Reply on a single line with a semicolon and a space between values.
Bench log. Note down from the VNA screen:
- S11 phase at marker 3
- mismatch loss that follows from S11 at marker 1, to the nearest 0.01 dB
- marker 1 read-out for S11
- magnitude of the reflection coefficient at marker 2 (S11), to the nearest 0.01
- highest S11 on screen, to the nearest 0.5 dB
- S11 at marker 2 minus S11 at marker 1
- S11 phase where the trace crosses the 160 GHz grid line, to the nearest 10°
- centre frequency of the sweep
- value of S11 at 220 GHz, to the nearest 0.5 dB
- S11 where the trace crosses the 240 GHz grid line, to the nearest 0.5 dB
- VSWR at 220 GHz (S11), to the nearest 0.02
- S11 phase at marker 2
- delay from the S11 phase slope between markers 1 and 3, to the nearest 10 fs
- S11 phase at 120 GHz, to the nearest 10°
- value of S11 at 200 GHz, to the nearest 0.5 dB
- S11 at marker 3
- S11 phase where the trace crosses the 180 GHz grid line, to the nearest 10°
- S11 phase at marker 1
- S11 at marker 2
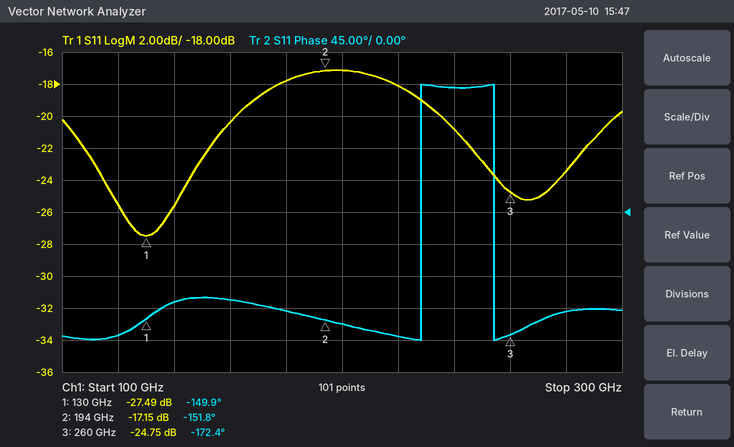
-172.4°; 0.01 dB; -27.49 dB; 0.14; -17.0 dB; 10.34 dB; -120°; 200 GHz; -18.0 dB; -21.0 dB; 1.28; -151.8°; 480 fs; -170°; -17.0 dB; -24.75 dB; -140°; -149.9°; -17.15 dB
